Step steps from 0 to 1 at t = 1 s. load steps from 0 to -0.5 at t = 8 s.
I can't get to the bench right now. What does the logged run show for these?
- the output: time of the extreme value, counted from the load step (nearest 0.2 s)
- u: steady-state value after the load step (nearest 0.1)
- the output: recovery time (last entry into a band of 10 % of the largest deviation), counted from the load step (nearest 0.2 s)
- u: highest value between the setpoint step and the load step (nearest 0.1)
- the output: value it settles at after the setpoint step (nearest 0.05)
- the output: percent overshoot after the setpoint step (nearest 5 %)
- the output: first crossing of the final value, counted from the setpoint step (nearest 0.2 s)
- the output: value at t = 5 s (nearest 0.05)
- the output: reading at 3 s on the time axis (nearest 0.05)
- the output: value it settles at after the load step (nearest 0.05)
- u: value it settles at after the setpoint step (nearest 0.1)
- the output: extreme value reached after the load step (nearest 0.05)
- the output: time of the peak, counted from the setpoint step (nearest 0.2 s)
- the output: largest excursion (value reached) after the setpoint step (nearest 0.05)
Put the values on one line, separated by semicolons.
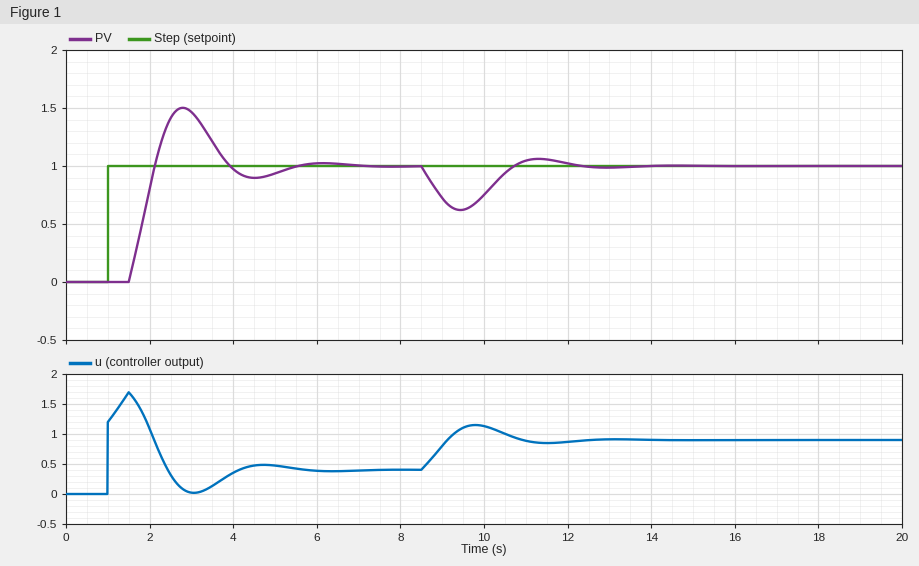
1.4 s; 0.9; 3.8 s; 1.7; 1.00; 50 %; 1.2 s; 0.95; 1.45; 1.00; 0.4; 0.60; 1.8 s; 1.50
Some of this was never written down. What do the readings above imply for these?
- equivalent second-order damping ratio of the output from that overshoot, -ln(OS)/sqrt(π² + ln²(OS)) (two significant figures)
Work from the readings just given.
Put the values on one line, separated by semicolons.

0.22
